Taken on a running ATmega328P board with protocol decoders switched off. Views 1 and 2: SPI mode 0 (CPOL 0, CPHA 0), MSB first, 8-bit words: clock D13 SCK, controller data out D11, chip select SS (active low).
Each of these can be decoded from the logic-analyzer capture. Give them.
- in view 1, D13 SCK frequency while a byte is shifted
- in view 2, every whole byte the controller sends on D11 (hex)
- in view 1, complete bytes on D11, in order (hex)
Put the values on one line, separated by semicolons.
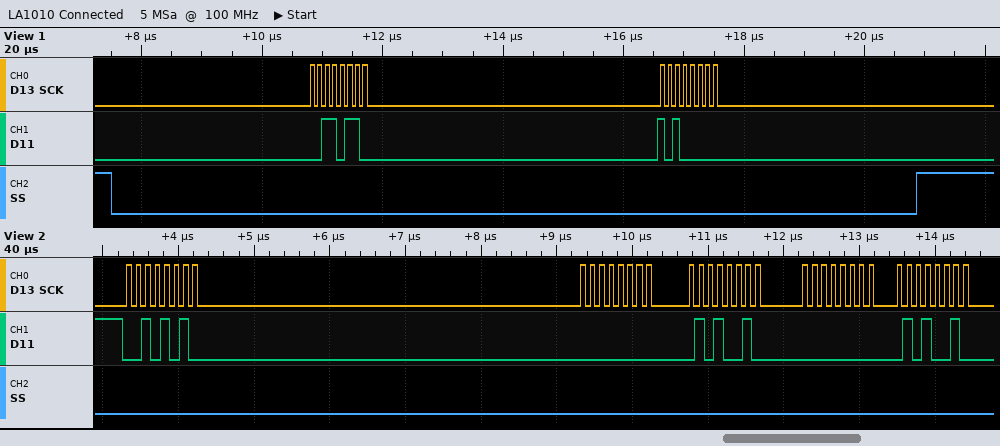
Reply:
8 MHz; 2A 00 52 00 52; 36 A0
